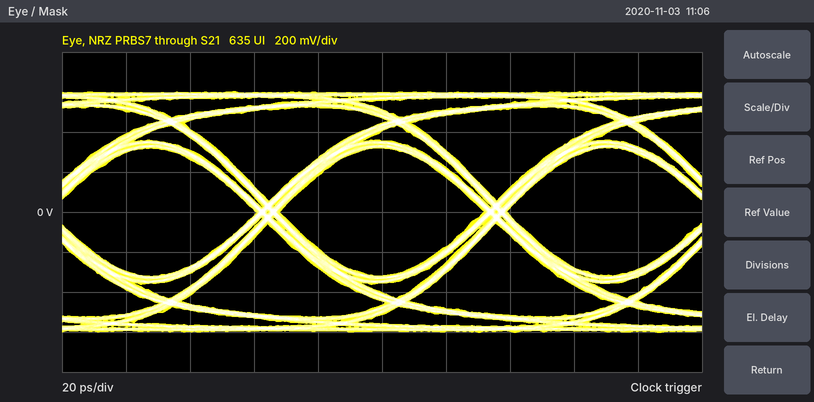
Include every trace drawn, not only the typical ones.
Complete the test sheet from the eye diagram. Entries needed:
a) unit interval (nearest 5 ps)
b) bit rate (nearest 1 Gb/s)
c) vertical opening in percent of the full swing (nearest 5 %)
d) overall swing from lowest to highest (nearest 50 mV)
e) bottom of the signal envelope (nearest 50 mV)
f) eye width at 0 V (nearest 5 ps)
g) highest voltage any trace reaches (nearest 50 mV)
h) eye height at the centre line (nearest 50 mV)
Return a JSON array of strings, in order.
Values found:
["70 ps", "14 Gb/s", "55 %", "1.20 V", "-600 mV", "65 ps", "600 mV", "650 mV"]
